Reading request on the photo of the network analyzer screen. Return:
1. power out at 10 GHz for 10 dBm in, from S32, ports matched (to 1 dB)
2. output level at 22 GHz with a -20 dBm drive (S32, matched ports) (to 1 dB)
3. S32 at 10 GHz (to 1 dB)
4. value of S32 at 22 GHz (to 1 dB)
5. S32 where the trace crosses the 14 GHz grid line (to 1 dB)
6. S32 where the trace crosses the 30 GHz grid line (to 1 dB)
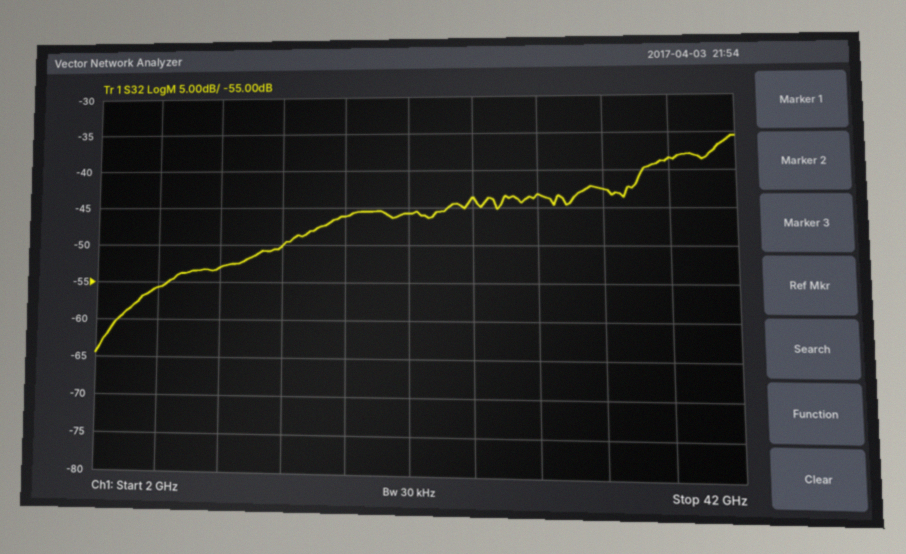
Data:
-43 dBm
-66 dBm
-53 dB
-46 dB
-50 dB
-43 dB
